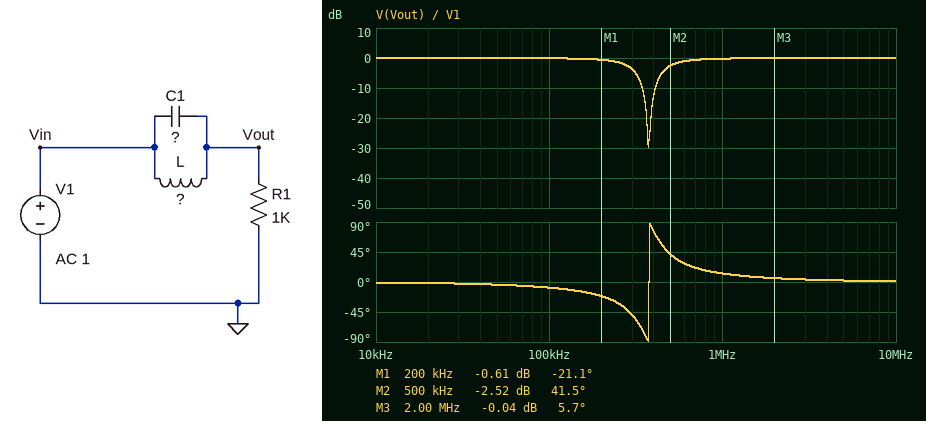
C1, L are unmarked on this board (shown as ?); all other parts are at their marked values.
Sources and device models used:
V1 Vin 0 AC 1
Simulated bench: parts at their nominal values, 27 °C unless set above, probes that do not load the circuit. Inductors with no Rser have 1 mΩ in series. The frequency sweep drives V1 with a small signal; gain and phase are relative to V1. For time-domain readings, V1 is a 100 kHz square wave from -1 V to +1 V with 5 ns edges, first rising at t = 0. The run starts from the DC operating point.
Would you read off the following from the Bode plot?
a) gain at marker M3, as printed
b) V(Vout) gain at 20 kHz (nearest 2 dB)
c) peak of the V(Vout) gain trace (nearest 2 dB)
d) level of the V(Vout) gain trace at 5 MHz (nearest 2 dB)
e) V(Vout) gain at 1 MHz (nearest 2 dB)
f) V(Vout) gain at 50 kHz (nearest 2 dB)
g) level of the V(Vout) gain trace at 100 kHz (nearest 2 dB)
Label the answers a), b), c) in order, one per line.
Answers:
a) -0.04 dB
b) 0 dB
c) 0 dB
d) 0 dB
e) 0 dB
f) 0 dB
g) 0 dB
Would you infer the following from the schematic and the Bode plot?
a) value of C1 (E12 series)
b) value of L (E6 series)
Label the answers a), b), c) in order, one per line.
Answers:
a) 820 pF
b) 220 µH
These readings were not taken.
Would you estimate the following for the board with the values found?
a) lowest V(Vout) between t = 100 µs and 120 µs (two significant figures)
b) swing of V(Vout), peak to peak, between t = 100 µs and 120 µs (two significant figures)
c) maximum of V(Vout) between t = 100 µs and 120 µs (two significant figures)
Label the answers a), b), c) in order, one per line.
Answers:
a) -1.3 V
b) 2.6 V
c) 1.3 V
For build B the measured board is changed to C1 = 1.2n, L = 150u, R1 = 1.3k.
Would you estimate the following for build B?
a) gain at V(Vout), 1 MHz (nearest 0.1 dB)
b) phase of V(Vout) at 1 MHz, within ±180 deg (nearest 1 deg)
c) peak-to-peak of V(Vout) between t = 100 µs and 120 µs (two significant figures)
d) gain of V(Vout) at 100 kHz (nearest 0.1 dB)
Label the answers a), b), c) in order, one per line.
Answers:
a) -0.1 dB
b) 7 deg
c) 2.5 V
d) 0 dB
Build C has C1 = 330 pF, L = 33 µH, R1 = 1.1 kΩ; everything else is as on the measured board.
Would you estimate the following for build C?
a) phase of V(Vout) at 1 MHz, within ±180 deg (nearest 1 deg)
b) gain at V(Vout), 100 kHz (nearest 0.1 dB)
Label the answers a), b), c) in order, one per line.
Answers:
a) -18 deg
b) 0 dB
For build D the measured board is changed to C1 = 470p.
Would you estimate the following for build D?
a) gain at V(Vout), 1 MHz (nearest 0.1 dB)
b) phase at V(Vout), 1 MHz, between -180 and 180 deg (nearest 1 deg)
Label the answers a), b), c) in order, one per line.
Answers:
a) -0.8 dB
b) 24 deg
